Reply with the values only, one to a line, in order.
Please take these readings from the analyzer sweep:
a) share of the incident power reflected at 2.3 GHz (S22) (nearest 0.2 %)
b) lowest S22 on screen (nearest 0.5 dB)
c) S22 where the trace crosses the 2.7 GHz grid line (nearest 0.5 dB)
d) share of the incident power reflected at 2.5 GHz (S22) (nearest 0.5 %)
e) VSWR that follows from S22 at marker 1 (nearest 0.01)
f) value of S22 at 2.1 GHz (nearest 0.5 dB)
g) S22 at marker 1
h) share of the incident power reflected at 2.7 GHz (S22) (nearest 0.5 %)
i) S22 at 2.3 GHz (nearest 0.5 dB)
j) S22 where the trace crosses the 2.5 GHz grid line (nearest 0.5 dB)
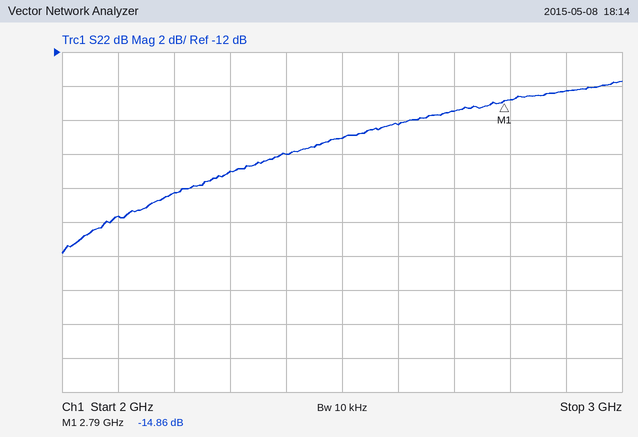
1.2 %
-24.0 dB
-15.5 dB
2.0 %
1.44
-21.5 dB
-14.86 dB
3.0 %
-19.0 dB
-17.0 dB
